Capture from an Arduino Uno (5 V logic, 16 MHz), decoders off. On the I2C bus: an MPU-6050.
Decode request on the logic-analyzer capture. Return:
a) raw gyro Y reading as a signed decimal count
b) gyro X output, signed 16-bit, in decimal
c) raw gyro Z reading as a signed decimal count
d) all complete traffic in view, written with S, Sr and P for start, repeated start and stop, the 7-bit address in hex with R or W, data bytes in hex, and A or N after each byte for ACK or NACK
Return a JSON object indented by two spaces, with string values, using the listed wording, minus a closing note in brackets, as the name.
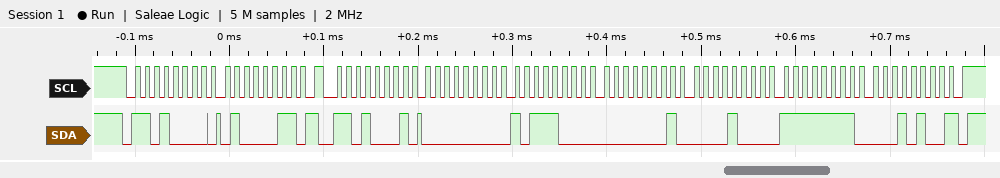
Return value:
{
  "raw gyro Y reading as a signed decimal count": "264",
  "gyro X output, signed 16-bit, in decimal": "184",
  "raw gyro Z reading as a signed decimal count": "-236",
  "all complete traffic in view, written with S, Sr and P for start, repeated start and stop, the 7-bit address in hex with R or W, data bytes in hex, and A or N after each byte for ACK or NACK": "S 68W A 43 A Sr 68R A 00 A B8 A 01 A 08 A FF A 14 N P"
}
